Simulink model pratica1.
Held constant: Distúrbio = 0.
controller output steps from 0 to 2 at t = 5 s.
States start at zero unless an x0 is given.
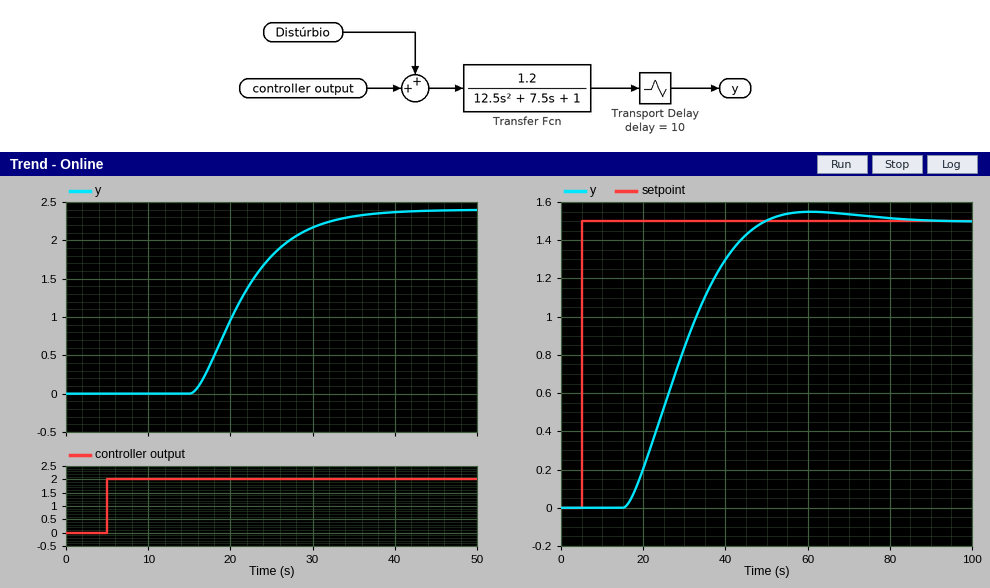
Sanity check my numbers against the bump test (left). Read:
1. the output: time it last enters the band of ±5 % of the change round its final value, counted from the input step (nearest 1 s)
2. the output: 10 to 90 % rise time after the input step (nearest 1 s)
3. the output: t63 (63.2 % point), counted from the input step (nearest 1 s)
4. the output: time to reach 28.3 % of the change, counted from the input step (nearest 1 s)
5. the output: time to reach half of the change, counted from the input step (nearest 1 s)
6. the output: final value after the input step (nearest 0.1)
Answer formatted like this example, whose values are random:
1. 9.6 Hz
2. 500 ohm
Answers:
1. 28 s
2. 13 s
3. 18 s
4. 14 s
5. 16 s
6. 2.4
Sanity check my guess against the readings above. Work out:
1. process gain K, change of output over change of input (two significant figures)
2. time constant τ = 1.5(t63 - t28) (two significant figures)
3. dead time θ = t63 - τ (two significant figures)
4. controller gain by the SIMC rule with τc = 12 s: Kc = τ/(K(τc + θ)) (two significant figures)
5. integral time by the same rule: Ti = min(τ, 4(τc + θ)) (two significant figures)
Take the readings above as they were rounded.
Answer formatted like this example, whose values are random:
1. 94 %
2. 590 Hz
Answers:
1. 1.2
2. 6.0 s
3. 12 s
4. 0.21
5. 6.0 s
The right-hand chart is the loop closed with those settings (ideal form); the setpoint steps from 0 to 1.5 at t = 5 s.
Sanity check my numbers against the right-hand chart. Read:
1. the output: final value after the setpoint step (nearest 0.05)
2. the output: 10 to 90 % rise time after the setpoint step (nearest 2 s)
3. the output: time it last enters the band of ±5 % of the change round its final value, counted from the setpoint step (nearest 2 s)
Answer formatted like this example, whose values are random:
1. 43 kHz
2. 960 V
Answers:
1. 1.50
2. 22 s
3. 40 s
